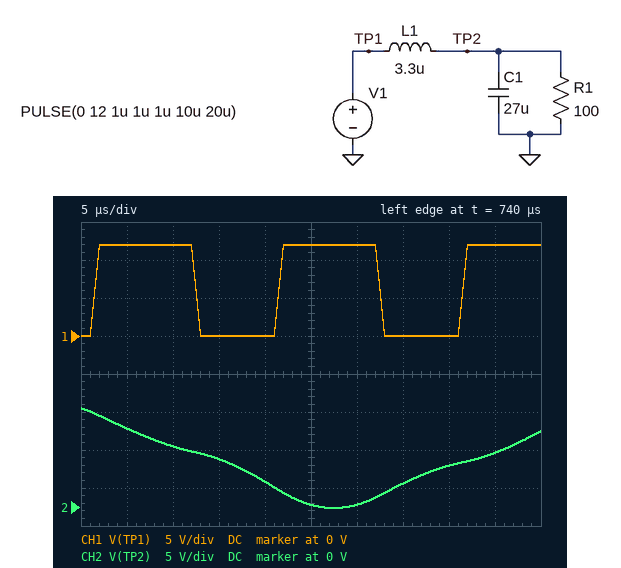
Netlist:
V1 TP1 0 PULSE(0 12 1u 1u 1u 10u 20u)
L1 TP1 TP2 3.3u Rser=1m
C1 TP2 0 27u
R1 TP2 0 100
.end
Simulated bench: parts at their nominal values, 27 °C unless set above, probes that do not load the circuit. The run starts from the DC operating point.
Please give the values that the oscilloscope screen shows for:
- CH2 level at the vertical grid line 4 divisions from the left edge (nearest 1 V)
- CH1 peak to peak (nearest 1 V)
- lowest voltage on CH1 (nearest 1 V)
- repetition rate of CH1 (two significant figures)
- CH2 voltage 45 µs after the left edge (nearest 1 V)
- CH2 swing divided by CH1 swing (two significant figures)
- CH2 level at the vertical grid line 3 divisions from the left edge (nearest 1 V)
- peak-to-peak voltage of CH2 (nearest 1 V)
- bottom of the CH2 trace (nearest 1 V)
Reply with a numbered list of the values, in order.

1. 3 V
2. 12 V
3. 0 V
4. 50 kHz
5. 7 V
6. 1.1
7. 6 V
8. 13 V
9. 0 V
